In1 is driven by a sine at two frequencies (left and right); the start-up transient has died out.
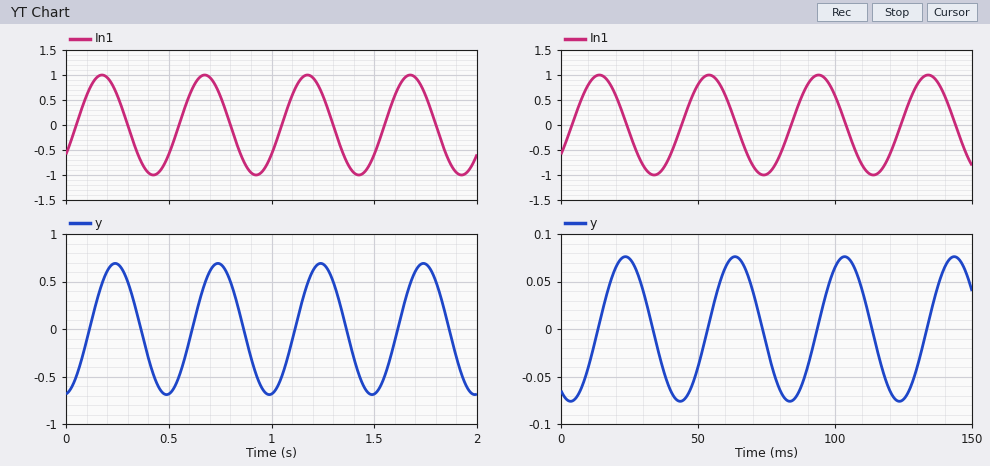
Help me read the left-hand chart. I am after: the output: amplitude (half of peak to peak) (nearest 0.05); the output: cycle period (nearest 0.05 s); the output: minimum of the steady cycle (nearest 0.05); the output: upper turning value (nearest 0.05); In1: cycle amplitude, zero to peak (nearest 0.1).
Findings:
0.70
0.50 s
-0.70
0.70
1.0
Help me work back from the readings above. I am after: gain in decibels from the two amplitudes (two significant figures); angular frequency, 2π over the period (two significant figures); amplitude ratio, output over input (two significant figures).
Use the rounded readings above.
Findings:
-3.1 dB
13 rad/s
0.70
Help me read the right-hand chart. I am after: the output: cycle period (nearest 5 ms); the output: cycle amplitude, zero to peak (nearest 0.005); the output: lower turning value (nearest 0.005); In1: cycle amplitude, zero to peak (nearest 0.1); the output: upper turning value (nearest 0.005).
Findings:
40 ms
0.075
-0.075
1.0
0.075
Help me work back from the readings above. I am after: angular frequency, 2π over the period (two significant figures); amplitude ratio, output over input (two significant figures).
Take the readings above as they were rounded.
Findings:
0.16 rad/ms
0.075
